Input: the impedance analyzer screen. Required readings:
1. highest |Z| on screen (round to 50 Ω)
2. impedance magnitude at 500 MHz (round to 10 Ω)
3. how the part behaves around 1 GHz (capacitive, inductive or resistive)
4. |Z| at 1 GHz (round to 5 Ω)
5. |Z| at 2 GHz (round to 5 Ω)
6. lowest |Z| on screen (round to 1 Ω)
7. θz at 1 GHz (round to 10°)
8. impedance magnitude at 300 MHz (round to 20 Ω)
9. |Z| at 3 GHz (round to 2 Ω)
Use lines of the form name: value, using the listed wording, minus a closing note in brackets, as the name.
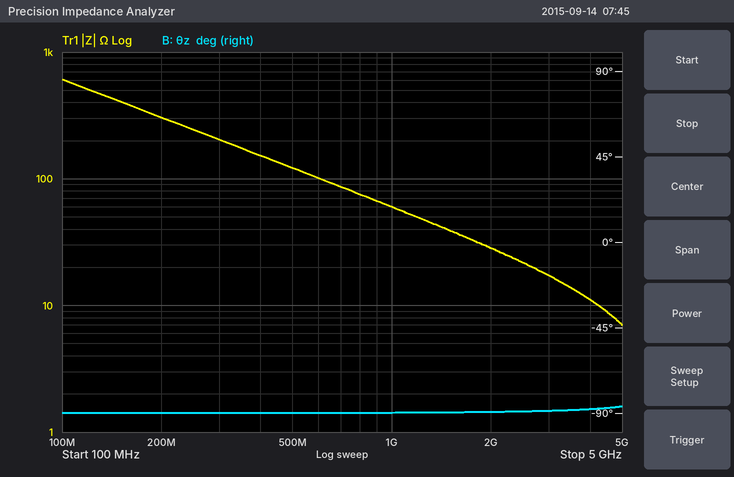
highest |Z| on screen: 600 Ω
impedance magnitude at 500 MHz: 120 Ω
how the part behaves around 1 GHz: capacitive
|Z| at 1 GHz: 60 Ω
|Z| at 2 GHz: 30 Ω
lowest |Z| on screen: 7 Ω
θz at 1 GHz: -90°
impedance magnitude at 300 MHz: 200 Ω
|Z| at 3 GHz: 18 Ω
